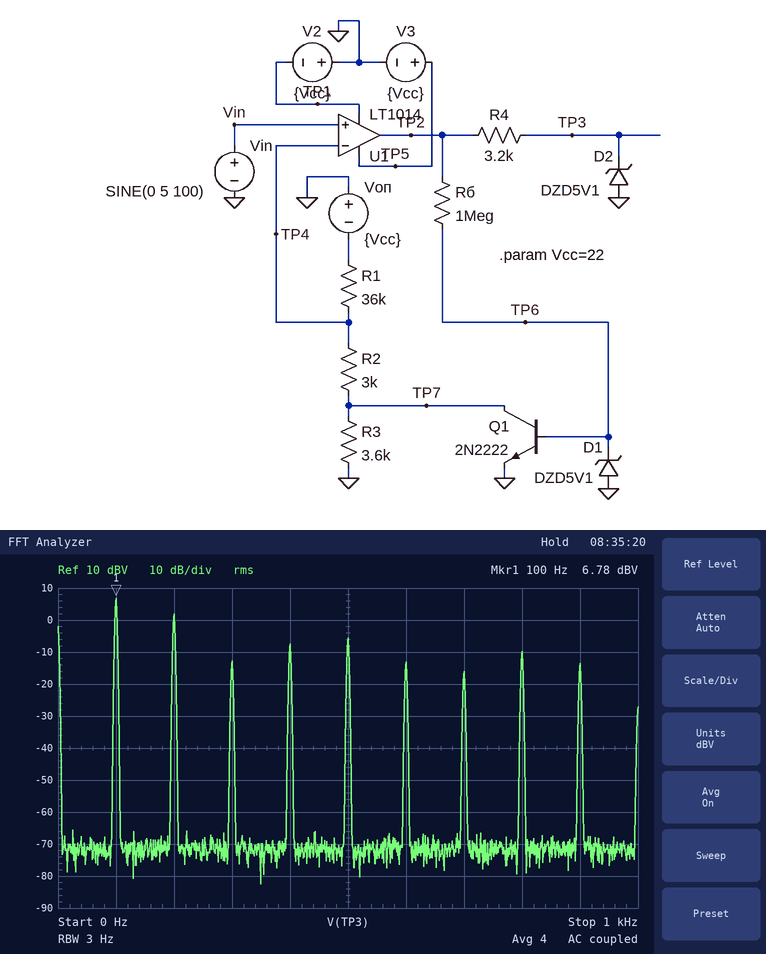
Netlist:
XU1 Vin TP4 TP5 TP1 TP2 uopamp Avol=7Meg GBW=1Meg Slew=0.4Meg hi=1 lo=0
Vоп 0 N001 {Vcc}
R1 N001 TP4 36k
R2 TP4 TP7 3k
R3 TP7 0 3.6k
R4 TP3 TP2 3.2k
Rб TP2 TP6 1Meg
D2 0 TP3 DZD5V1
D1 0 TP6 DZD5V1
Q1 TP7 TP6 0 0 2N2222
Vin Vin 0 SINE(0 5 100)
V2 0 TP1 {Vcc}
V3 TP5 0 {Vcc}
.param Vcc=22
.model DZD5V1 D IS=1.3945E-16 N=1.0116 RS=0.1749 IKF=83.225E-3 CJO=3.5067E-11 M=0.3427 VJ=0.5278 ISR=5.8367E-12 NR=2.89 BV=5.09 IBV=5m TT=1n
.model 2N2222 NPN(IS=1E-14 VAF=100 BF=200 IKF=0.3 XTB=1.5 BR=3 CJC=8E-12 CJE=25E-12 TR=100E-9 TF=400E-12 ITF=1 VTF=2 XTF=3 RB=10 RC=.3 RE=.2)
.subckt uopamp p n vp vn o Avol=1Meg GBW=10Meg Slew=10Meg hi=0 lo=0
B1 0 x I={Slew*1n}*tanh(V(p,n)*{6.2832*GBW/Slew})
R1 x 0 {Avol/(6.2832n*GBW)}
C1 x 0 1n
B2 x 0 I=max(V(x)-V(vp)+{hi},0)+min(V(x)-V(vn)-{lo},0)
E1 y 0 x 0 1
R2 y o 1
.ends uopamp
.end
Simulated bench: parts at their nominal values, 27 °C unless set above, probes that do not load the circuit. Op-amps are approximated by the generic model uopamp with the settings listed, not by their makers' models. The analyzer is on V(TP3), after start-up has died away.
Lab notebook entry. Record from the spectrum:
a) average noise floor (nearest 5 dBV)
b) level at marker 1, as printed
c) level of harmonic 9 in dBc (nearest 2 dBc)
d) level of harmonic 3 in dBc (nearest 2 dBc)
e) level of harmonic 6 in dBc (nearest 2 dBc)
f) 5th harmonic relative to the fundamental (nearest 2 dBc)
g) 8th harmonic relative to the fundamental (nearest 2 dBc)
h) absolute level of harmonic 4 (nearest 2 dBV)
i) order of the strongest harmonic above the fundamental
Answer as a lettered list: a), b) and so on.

a) -70 dBV
b) 6.78 dBV
c) -20 dBc
d) -20 dBc
e) -20 dBc
f) -12 dBc
g) -16 dBc
h) -8 dBV
i) 2
